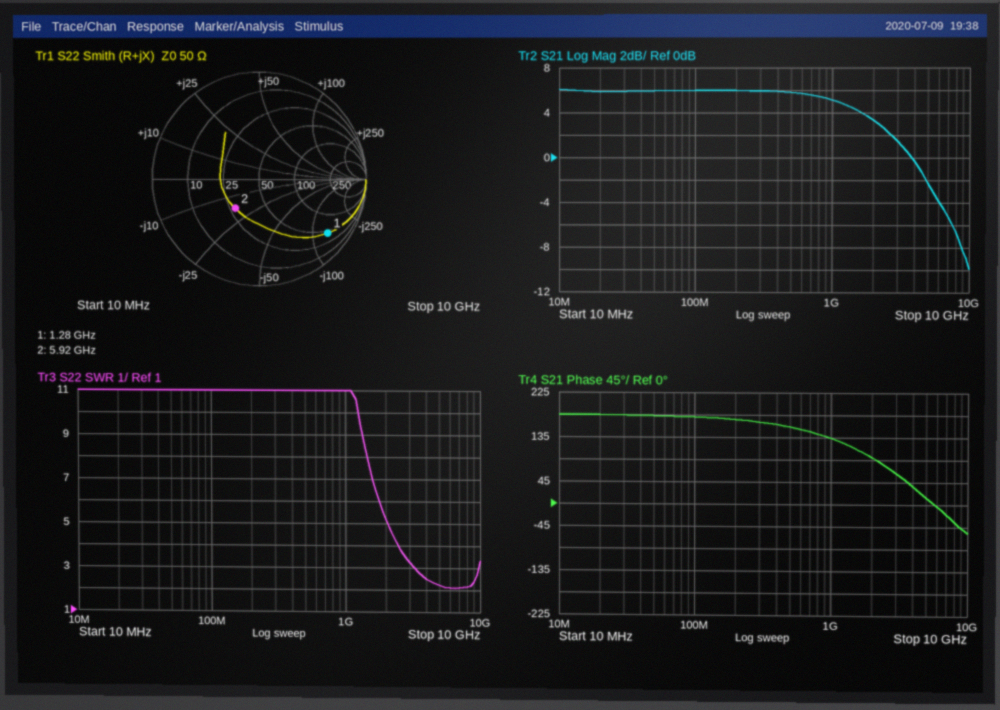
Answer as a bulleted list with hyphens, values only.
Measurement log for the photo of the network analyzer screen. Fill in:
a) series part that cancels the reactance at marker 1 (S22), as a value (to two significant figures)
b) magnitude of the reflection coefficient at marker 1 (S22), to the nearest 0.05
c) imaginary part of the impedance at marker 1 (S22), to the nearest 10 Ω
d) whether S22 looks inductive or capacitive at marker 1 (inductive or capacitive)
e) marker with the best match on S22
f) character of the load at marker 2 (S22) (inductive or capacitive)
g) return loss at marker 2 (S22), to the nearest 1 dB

- 16 nH
- 0.80
- -130 Ω
- capacitive
- marker 2
- capacitive
- 9 dB
